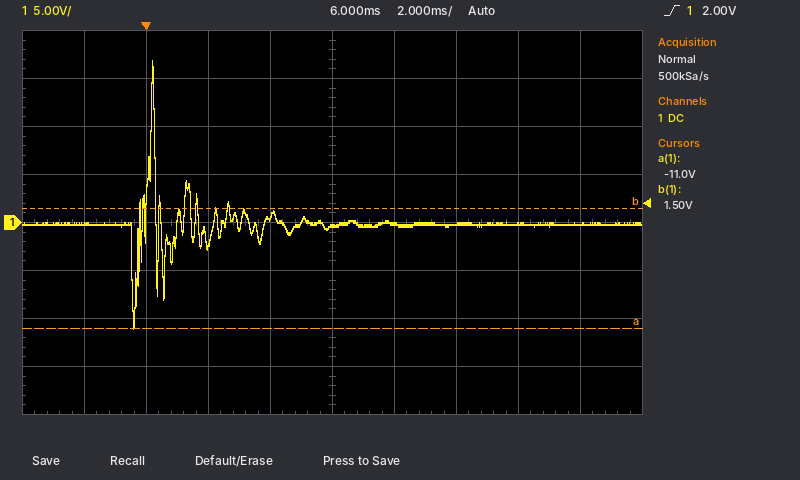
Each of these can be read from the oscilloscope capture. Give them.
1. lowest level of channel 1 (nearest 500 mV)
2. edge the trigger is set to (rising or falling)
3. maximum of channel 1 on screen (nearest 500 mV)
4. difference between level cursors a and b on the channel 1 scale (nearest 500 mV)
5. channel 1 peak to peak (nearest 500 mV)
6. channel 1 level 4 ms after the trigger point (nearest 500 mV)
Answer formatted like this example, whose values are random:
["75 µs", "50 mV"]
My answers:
["-11.0 V", "rising", "17.0 V", "12.5 V", "28.0 V", "500 mV"]
